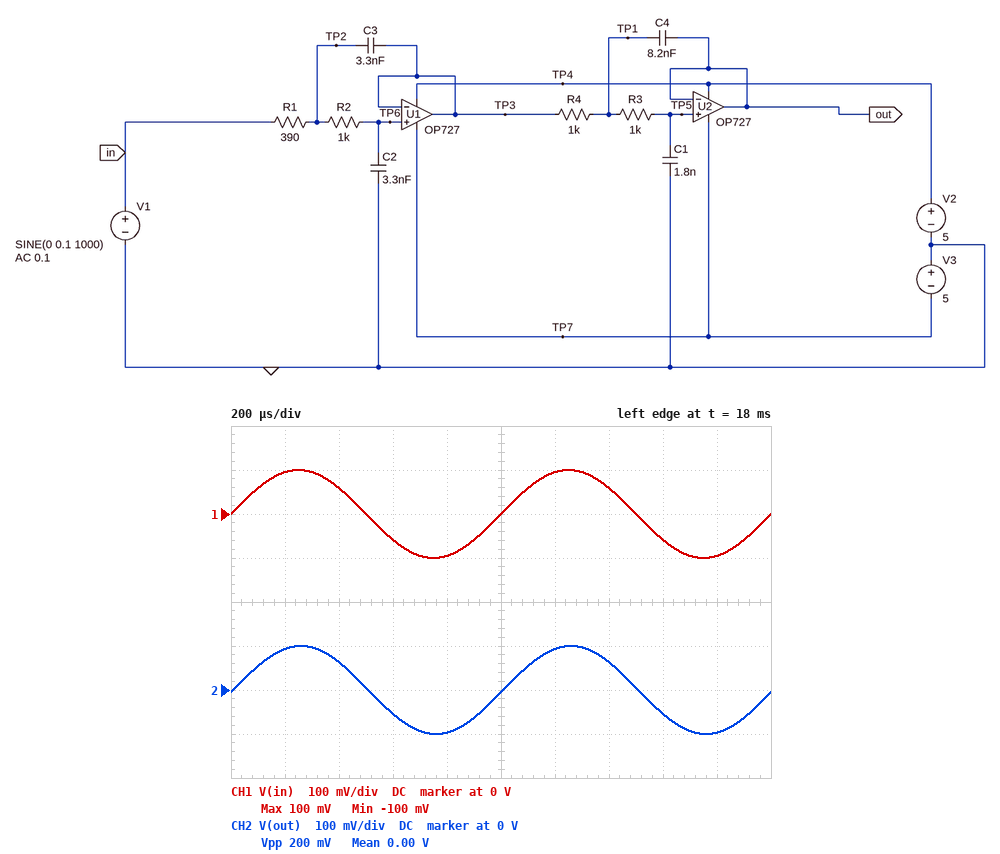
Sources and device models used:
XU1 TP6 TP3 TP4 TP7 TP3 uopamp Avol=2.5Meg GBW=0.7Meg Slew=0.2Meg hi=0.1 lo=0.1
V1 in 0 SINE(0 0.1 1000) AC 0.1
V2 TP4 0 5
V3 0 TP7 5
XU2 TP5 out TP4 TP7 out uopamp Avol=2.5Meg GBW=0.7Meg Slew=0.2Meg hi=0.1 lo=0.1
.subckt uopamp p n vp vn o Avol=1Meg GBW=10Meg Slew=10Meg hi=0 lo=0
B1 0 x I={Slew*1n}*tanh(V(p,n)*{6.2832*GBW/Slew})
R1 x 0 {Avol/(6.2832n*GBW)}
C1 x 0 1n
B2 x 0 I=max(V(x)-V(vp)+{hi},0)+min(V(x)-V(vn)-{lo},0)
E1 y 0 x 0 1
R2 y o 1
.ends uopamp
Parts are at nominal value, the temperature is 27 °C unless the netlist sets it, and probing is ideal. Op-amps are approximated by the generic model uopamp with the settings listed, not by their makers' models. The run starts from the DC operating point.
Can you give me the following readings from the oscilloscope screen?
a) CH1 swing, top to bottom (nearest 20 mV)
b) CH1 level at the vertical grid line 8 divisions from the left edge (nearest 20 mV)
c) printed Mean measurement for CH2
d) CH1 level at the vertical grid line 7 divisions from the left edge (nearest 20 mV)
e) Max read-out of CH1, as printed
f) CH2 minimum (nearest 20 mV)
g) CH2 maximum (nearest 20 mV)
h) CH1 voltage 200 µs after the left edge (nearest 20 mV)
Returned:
200 mV
-60 mV
0.00 V
60 mV
100 mV
-100 mV
100 mV
100 mV
